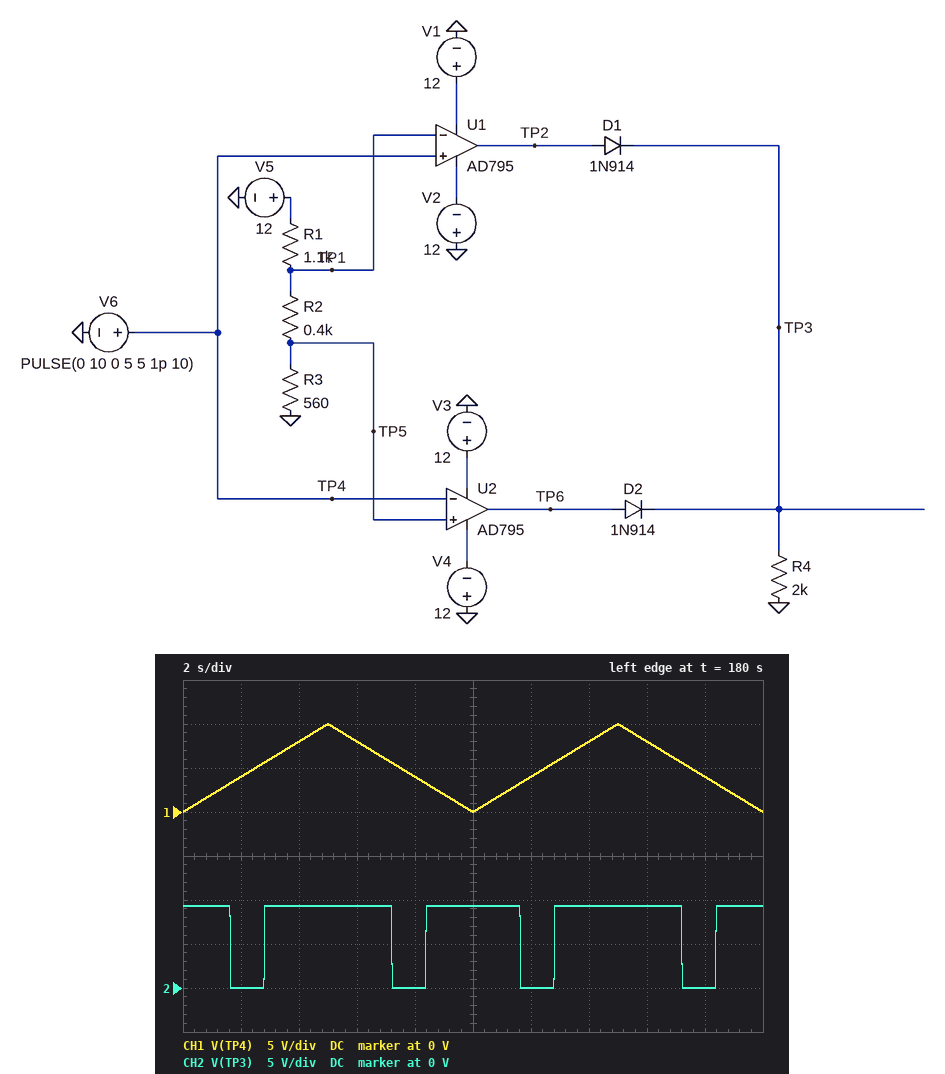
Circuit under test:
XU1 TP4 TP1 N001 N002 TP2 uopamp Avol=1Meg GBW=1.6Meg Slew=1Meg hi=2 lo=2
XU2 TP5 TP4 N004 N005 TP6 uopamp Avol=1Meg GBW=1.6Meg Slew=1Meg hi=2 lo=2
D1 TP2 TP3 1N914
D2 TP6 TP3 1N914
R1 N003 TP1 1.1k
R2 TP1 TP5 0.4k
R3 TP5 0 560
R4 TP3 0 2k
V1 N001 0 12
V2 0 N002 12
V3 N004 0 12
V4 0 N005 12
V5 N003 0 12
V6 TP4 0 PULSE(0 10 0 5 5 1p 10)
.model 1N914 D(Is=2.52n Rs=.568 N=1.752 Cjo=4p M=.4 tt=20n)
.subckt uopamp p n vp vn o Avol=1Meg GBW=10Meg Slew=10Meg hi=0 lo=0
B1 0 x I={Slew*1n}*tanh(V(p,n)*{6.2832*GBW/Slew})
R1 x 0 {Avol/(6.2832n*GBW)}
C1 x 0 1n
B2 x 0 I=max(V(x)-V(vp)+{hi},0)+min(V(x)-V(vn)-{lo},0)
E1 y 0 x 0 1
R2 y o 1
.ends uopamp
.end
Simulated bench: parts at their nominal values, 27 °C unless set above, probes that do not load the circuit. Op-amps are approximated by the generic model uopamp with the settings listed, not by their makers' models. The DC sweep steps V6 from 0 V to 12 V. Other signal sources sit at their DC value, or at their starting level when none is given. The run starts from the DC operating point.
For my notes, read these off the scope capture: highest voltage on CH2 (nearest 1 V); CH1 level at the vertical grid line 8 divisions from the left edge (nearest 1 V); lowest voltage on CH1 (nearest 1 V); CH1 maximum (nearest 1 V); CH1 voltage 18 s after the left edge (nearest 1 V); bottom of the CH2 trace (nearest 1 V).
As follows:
9 V
8 V
0 V
10 V
4 V
0 V
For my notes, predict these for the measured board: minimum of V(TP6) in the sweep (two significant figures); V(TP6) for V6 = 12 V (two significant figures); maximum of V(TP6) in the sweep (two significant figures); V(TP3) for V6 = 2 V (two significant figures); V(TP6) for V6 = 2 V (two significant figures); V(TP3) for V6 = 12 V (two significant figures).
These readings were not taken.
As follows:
-10 V
-10 V
10 V
9.3 V
10 V
9.3 V
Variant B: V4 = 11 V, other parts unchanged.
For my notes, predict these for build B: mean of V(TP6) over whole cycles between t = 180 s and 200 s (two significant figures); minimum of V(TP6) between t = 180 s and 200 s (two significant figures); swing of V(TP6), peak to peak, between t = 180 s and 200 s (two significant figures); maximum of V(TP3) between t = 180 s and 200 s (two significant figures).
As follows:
-2.8 V
-9.0 V
19 V
9.3 V
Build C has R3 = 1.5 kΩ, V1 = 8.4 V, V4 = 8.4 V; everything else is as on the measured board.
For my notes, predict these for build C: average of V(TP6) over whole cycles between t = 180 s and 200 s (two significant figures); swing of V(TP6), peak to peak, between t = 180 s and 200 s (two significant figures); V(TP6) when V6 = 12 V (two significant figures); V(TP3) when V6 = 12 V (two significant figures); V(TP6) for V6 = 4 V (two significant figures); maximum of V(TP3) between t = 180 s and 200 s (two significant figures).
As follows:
3.4 V
16 V
-6.4 V
5.8 V
10 V
9.3 V
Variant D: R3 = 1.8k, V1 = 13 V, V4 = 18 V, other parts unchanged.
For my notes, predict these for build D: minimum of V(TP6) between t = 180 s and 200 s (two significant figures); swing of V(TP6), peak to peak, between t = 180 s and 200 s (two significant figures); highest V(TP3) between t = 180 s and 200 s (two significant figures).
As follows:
-16 V
26 V
10 V
